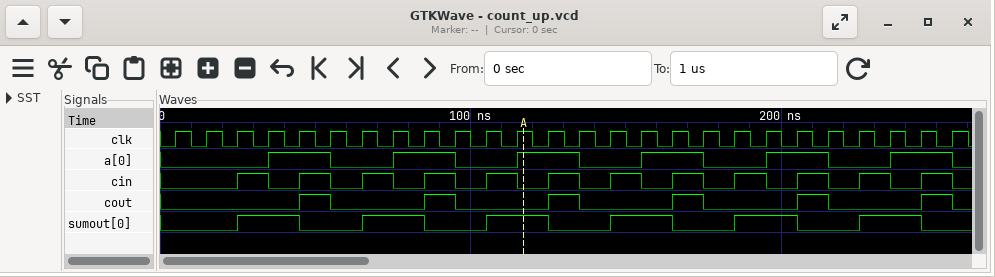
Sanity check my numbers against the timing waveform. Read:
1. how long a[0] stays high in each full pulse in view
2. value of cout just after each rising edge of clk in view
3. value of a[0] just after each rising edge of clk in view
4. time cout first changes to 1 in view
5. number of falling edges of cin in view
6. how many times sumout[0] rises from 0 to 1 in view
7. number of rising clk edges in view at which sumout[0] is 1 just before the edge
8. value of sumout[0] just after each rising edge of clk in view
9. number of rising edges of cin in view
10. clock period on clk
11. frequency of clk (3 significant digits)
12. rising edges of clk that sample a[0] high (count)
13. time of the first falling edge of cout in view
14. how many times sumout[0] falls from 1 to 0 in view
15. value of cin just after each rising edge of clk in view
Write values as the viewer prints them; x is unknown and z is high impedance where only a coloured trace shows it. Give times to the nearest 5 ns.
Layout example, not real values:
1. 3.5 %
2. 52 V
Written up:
1. 20 ns, 20 ns, 20 ns, 20 ns, 20 ns, 20 ns
2. 0 0 0 0 1 0 0 0 1 0 0 0 1 0 0 0 1 0 0 0 1 0 0 0 1 0
3. 0 0 0 1 1 0 0 1 1 0 0 1 1 0 0 1 1 0 0 1 1 0 0 1 1 0
4. 45 ns
5. 12
6. 6
7. 12
8. 0 0 1 1 0 0 1 1 0 0 1 1 0 0 1 1 0 0 1 1 0 0 1 1 0 0
9. 12
10. 10 ns
11. 100 MHz
12. 12
13. 55 ns
14. 6
15. 0 0 1 0 1 0 1 0 1 0 1 0 1 0 1 0 1 0 1 0 1 0 1 0 1 0
